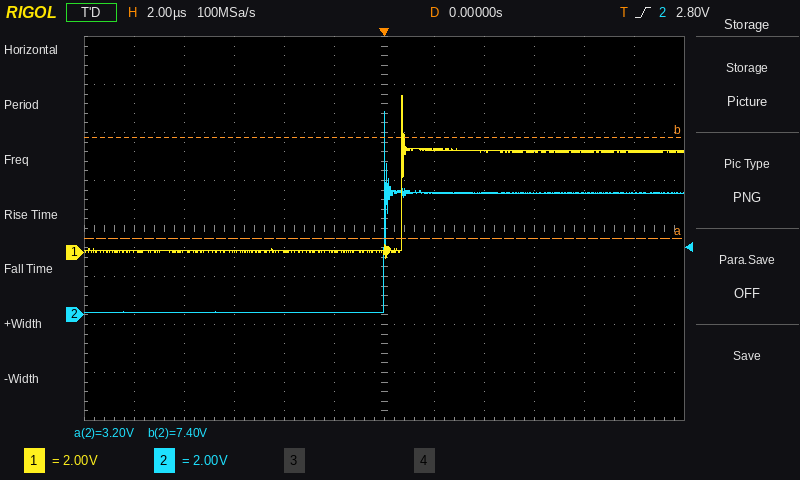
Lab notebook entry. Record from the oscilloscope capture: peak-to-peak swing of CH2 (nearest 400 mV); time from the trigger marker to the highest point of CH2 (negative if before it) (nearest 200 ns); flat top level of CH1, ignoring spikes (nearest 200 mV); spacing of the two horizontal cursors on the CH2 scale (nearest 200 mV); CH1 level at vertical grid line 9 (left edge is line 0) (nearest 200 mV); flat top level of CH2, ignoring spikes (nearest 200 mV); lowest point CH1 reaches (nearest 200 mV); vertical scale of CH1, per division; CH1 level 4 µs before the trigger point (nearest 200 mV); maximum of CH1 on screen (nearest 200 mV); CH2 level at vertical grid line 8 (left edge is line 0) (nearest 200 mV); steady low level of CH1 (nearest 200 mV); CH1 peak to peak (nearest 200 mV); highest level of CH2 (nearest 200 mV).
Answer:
8.4 V
0.0 µs
4.2 V
4.2 V
4.2 V
5.0 V
-200 mV
2 V
0.0 V
6.6 V
5.0 V
0.0 V
6.8 V
8.4 V
